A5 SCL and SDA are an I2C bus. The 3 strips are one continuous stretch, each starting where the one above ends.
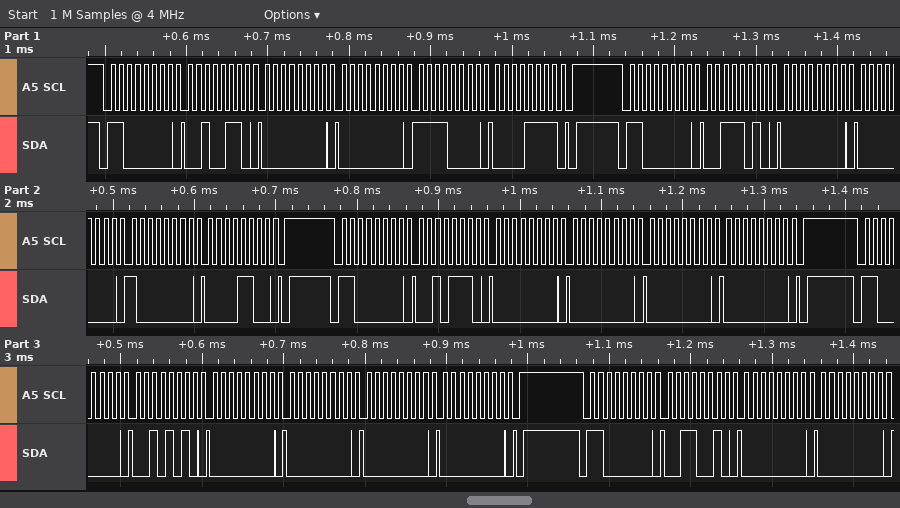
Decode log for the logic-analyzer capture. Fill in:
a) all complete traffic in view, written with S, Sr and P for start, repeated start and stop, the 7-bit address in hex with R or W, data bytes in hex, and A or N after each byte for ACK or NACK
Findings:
S 60W A 26 A 00 A 00 A F0 A 0F A P S 60W A 3A A 00 A 00 A 80 A 0C A P S 60W A 2E A 00 A 00 A 00 A 00 A P S 60W A 2A A 00 A 00 A 00 A 00 A P S 60W A 32 A 00 A 00 A
